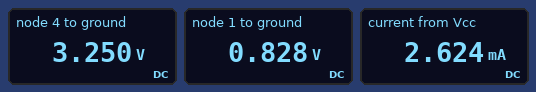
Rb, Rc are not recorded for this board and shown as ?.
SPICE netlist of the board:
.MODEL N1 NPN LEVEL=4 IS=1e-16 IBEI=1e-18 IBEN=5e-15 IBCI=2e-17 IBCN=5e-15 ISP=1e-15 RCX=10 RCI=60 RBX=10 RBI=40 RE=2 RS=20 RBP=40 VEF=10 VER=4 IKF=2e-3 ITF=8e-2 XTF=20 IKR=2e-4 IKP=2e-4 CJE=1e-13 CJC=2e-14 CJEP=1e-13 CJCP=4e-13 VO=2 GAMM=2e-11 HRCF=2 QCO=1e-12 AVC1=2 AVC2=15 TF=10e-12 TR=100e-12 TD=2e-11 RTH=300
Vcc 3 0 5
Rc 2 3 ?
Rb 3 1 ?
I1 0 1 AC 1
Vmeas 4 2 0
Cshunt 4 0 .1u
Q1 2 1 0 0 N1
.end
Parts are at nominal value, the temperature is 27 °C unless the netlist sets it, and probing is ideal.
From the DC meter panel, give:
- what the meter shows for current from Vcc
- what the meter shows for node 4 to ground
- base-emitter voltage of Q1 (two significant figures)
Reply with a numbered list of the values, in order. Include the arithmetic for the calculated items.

1. 2.624 mA
2. 3.250 V
3. 828 mV = 830 mV
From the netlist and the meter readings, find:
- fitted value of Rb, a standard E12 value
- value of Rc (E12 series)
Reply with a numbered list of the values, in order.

1. 82 kΩ
2. 680 Ω
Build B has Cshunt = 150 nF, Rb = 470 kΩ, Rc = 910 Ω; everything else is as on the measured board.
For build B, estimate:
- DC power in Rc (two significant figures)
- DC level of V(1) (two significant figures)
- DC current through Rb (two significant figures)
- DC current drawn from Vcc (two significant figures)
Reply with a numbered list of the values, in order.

1. 1.8 mW
2. 800 mV
3. 8.9 µA
4. 1.4 mA
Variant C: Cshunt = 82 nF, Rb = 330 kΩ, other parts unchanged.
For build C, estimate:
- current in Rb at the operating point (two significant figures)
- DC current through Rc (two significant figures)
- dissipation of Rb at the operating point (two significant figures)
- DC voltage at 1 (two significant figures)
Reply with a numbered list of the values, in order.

1. 13 µA
2. 1.8 mA
3. 53 µW
4. 810 mV
